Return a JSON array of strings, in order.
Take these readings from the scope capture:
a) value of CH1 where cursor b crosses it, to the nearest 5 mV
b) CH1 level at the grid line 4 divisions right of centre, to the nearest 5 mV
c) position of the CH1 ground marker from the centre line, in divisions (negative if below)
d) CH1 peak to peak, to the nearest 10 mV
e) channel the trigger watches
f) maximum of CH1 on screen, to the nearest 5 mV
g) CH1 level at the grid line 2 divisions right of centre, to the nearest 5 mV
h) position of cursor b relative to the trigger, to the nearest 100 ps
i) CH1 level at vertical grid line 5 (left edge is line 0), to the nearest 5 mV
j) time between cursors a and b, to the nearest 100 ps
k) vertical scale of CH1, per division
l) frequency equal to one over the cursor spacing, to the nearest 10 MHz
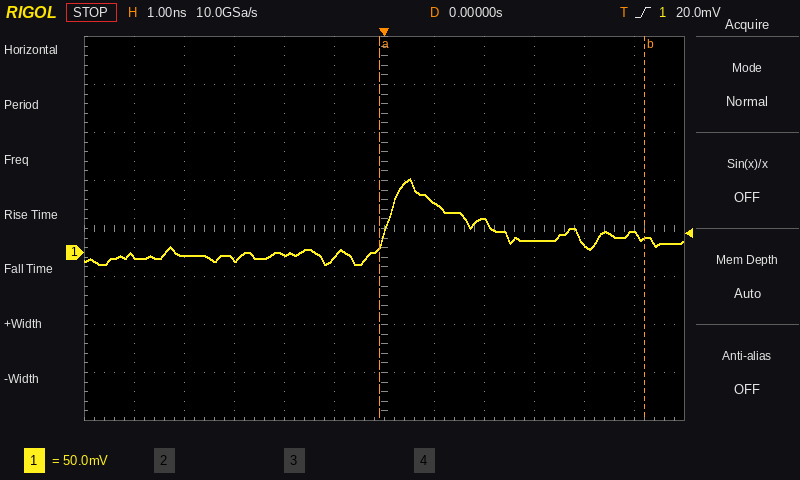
["15 mV", "10 mV", "-0.5 div", "90 mV", "CH1", "75 mV", "35 mV", "+5.2 ns", "-5 mV", "5.3 ns", "50 mV", "190 MHz"]
